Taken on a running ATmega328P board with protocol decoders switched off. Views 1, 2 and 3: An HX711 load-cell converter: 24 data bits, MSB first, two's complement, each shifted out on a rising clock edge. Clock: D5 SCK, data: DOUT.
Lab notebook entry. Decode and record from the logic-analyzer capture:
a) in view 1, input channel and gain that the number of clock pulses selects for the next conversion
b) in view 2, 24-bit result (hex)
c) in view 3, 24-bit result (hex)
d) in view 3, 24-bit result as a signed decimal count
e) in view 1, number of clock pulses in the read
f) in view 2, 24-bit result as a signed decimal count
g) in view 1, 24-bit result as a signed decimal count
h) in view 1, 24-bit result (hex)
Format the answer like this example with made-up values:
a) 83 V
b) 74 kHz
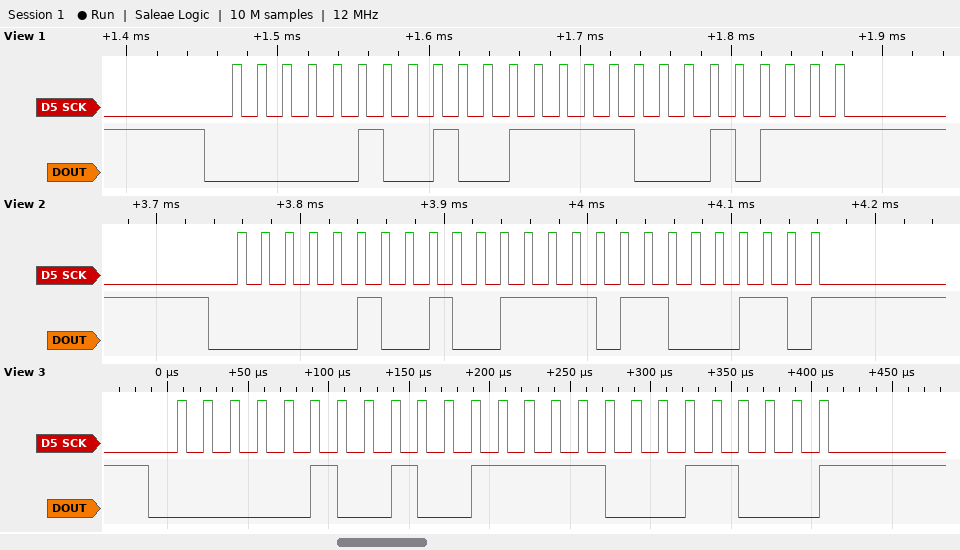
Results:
a) channel A, gain 128
b) 0x049EC6
c) 0x049F18
d) 302872
e) 25
f) 302790
g) 302871
h) 0x049F17
